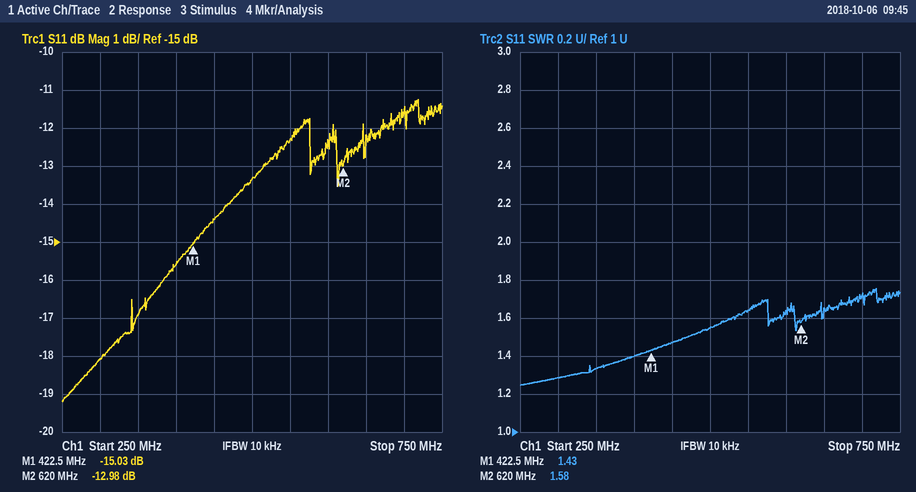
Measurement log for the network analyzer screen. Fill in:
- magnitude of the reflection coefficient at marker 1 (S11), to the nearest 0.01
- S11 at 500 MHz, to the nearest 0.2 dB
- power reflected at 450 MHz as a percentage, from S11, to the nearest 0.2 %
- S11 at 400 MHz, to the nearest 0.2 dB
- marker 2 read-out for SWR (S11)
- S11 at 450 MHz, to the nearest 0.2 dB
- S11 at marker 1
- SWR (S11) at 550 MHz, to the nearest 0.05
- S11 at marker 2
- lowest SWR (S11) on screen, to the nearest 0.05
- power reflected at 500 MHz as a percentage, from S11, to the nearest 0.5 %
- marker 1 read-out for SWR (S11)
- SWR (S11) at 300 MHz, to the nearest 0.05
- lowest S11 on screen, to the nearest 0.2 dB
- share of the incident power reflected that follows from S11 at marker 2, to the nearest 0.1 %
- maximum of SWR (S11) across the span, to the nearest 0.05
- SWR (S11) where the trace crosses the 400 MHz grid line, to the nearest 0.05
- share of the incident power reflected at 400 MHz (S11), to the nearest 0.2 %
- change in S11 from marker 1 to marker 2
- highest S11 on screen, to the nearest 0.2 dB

0.18
-13.4 dB
3.6 %
-15.6 dB
1.58
-14.4 dB
-15.03 dB
1.65
-12.98 dB
1.25
4.5 %
1.43
1.30
-19.2 dB
5.0 %
1.75
1.40
2.8 %
2.05 dB
-11.2 dB
